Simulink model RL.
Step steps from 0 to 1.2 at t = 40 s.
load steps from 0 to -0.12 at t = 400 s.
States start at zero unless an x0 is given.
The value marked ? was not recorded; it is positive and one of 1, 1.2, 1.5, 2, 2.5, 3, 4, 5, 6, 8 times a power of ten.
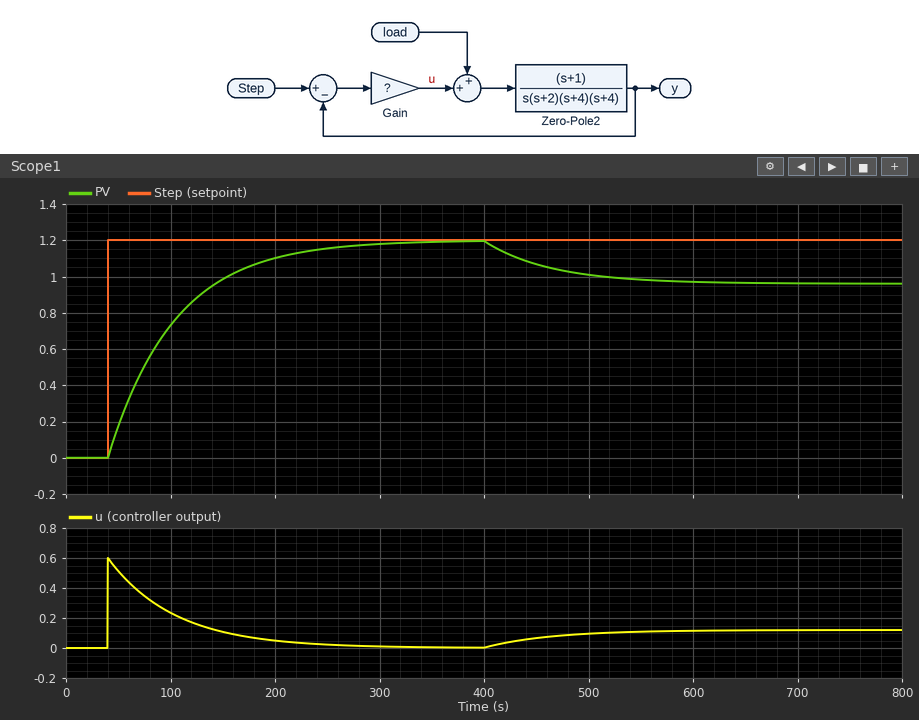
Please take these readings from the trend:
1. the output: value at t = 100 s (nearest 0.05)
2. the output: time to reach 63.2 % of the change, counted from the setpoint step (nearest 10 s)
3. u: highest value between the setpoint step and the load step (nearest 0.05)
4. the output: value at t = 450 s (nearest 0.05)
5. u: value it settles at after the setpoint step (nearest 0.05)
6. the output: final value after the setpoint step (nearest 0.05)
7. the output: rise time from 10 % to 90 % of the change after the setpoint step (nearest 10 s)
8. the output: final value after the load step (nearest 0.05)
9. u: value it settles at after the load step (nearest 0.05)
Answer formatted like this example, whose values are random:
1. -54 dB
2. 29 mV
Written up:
1. 0.75
2. 60 s
3. 0.60
4. 1.05
5. 0.00
6. 1.20
7. 140 s
8. 0.95
9. 0.10
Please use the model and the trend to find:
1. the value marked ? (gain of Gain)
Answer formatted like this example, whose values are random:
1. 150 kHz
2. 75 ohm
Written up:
1. 0.5
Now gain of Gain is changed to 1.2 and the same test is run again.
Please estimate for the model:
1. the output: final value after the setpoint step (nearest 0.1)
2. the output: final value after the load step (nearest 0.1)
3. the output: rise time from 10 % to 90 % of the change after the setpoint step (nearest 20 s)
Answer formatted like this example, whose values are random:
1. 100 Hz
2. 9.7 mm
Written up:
1. 1.2
2. 1.1
3. 60 s
